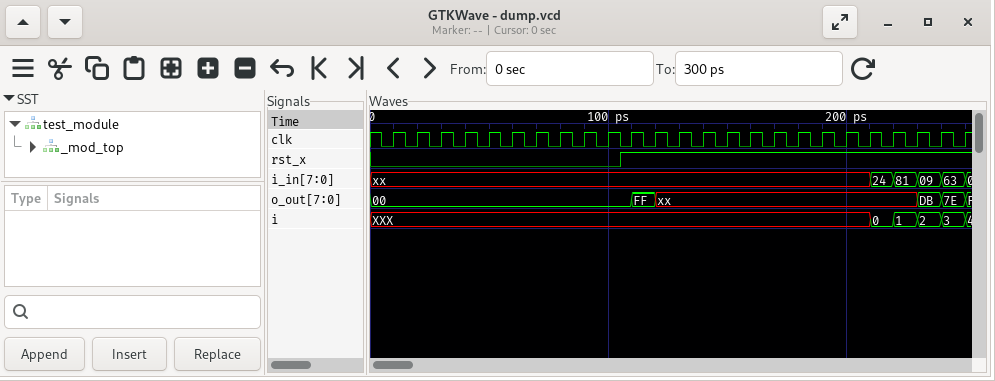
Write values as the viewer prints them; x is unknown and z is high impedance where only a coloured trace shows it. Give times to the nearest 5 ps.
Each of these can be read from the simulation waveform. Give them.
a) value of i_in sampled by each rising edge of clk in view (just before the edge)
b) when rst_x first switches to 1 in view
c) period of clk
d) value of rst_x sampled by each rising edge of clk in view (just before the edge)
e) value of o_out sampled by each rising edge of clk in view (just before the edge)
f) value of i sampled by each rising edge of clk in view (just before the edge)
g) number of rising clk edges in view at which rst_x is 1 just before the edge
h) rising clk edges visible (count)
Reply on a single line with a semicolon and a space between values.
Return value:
xx, xx, xx, xx, xx, xx, xx, xx, xx, xx, xx, xx, xx, xx, xx, xx, xx, xx, xx, xx, xx, 24, 81, 09, 63; 105 ps; 10 ps; 0 0 0 0 0 0 0 0 0 0 1 1 1 1 1 1 1 1 1 1 1 1 1 1 1; 00, 00, 00, 00, 00, 00, 00, 00, 00, 00, 00, FF, xx, xx, xx, xx, xx, xx, xx, xx, xx, xx, xx, DB, 7E; XXX, XXX, XXX, XXX, XXX, XXX, XXX, XXX, XXX, XXX, XXX, XXX, XXX, XXX, XXX, XXX, XXX, XXX, XXX, XXX, XXX, 0, 1, 2, 3; 15; 25
